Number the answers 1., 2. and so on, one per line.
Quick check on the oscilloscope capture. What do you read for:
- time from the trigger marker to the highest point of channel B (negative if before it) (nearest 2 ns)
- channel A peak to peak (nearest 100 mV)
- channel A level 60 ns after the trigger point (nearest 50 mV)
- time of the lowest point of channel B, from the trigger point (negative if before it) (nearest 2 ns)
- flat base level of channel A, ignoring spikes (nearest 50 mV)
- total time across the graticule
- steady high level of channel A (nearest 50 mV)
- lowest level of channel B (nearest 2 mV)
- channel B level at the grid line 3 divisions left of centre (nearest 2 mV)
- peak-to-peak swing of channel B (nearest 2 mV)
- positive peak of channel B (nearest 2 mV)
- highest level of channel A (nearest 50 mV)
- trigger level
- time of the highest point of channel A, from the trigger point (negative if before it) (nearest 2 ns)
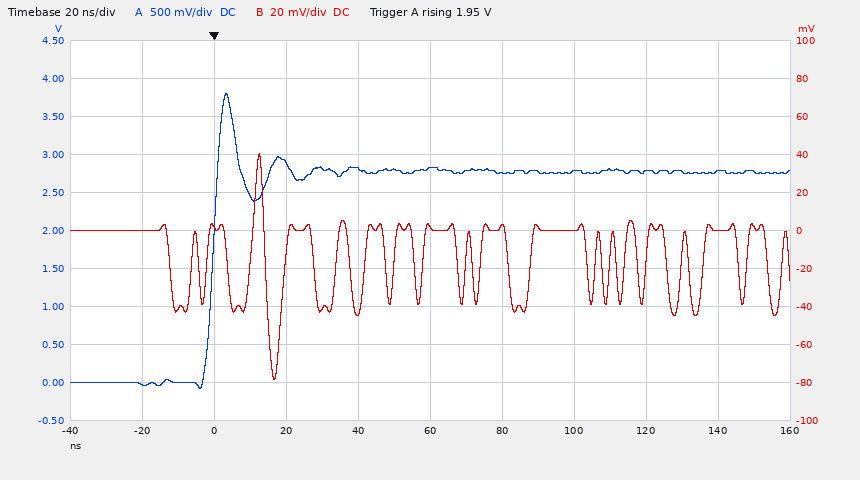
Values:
1. +12 ns
2. 3.90 V
3. 2.80 V
4. +16 ns
5. 0 mV
6. 200 ns
7. 2.75 V
8. -78 mV
9. 2 mV
10. 118 mV
11. 40 mV
12. 3.80 V
13. 1.95 V
14. +4 ns
